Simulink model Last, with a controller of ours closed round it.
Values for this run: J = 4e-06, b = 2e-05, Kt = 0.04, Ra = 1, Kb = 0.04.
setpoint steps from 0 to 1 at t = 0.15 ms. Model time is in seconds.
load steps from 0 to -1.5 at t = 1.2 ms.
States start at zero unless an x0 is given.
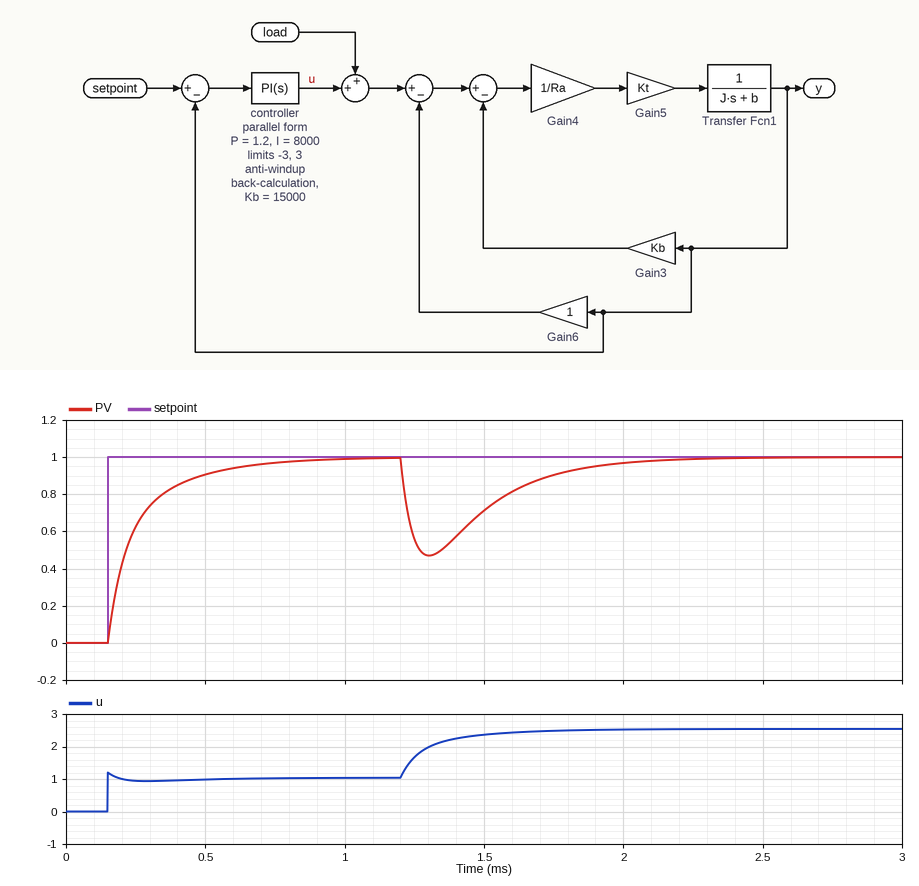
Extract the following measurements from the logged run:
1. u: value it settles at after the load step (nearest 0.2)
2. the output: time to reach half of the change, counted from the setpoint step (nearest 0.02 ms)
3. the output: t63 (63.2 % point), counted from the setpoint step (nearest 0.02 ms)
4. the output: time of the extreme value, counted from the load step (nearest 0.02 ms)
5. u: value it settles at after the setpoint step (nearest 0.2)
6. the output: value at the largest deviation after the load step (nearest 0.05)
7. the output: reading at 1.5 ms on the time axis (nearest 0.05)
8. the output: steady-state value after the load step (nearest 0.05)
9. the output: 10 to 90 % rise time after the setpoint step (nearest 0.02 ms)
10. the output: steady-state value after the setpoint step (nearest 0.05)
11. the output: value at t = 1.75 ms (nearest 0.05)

2.6
0.06 ms
0.10 ms
0.10 ms
1.0
0.45
0.70
1.00
0.32 ms
1.00
0.90
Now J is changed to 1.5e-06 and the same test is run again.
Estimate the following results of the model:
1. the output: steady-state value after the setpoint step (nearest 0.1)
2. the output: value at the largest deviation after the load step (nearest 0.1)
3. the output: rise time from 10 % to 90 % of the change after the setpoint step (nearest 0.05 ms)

1.0
0.4
0.40 ms
